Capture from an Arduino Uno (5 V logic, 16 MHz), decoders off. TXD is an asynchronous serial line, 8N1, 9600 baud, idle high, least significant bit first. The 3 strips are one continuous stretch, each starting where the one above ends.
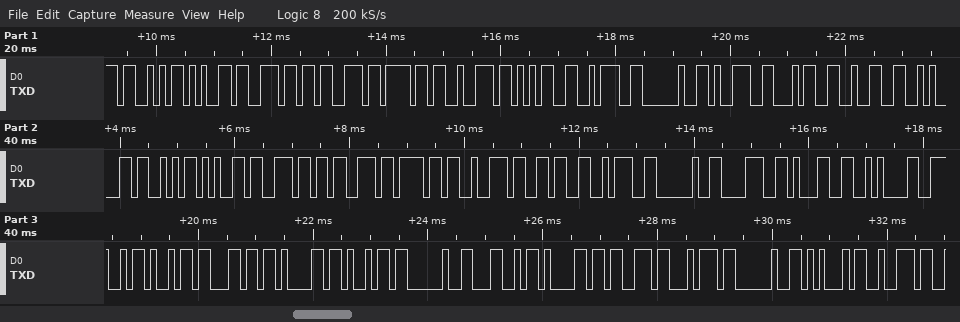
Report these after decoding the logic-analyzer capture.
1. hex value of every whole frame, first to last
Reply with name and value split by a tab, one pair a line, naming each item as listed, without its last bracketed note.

hex value of every whole frame, first to last	53 65 6E 73 6F 72 35 3A 20 39 34 32 0A 53 65 6E 73 6F 72 36 3A 20 38 31 0A 4E 69 6C 61 69 20 4C 61 73 74 20 45 72
